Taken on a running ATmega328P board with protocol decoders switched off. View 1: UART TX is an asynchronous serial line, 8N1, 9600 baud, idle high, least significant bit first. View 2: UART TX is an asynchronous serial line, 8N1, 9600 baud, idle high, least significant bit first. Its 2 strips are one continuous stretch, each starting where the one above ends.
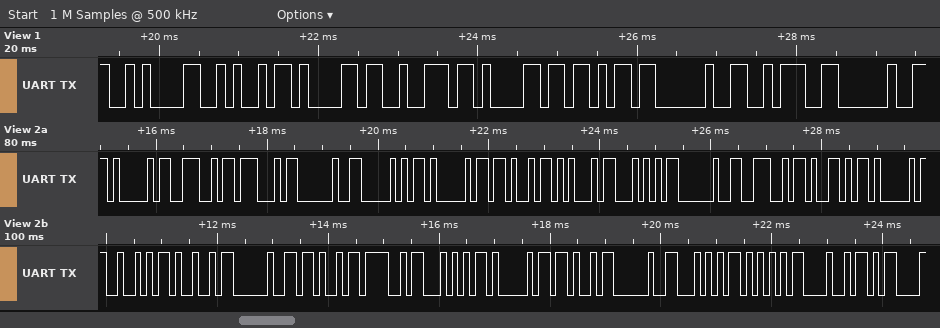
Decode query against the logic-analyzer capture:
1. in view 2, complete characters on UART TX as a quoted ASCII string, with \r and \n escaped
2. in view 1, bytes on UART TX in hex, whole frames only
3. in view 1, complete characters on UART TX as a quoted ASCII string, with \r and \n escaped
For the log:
"ANG PAKET NYARI KOTAK TUH\r"
0A 4A 61 72 61 6B 20 3A 20
"\nJarak : "
